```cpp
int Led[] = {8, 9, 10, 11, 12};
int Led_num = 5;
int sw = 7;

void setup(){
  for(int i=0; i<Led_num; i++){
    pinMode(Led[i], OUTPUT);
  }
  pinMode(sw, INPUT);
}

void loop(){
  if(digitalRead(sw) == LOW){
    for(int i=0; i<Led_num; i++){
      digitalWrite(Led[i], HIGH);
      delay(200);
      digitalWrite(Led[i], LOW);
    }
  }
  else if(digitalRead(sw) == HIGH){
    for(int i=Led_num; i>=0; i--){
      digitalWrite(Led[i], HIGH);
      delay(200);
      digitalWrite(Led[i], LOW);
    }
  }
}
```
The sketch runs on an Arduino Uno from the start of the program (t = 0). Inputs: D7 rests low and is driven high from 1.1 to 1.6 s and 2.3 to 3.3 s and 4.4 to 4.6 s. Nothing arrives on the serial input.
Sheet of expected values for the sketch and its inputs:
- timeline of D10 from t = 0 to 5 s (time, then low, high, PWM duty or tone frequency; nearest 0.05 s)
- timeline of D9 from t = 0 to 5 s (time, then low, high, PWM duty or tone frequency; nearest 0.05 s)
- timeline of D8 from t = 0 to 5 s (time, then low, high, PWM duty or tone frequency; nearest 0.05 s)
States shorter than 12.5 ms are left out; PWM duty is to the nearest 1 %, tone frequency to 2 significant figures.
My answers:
0 s low; 0.4 s high; 0.6 s low; 1.4 s high; 1.6 s low; 2.4 s high; 2.6 s low; 3.6 s high; 3.8 s low; 4.6 s high; 4.8 s low
0 s low; 0.2 s high; 0.4 s low; 1.2 s high; 1.4 s low; 2.2 s high; 2.4 s low; 3.8 s high; 4 s low; 4.4 s high; 4.6 s low
0 s high; 0.2 s low; 1 s high; 1.2 s low; 2 s high; 2.2 s low; 4 s high; 4.4 s low
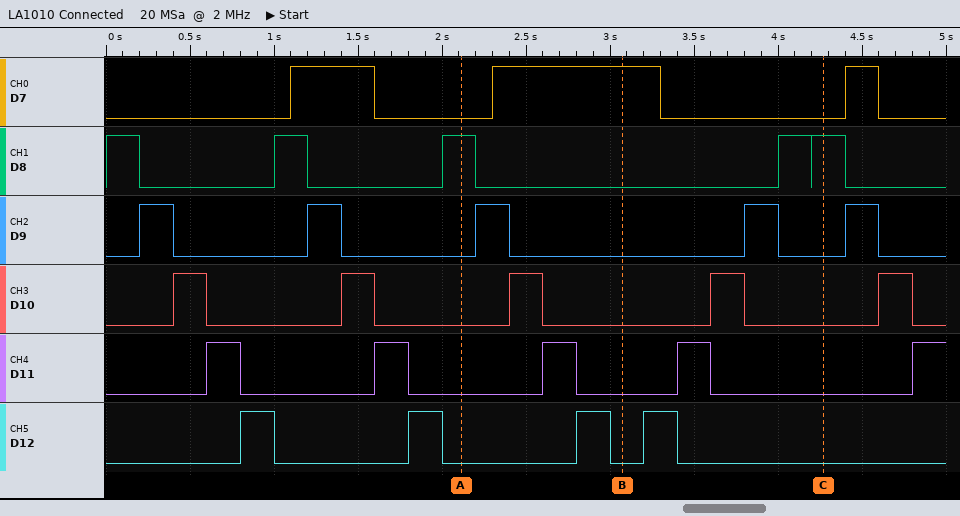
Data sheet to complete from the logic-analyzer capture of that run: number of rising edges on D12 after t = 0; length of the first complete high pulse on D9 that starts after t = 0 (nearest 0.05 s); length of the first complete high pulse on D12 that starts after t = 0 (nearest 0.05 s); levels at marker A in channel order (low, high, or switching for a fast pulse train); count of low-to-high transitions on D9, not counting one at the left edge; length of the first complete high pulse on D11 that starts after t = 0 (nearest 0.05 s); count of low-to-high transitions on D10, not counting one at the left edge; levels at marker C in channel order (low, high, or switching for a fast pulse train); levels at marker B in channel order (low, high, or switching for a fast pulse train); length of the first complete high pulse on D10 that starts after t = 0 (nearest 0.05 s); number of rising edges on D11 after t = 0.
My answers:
4
0.20 s
0.20 s
D7 low, D8 high, D9 low, D10 low, D11 low, D12 low
5
0.20 s
5
D7 low, D8 high, D9 low, D10 low, D11 low, D12 low
D7 high, D8 low, D9 low, D10 low, D11 low, D12 low
0.20 s
5
